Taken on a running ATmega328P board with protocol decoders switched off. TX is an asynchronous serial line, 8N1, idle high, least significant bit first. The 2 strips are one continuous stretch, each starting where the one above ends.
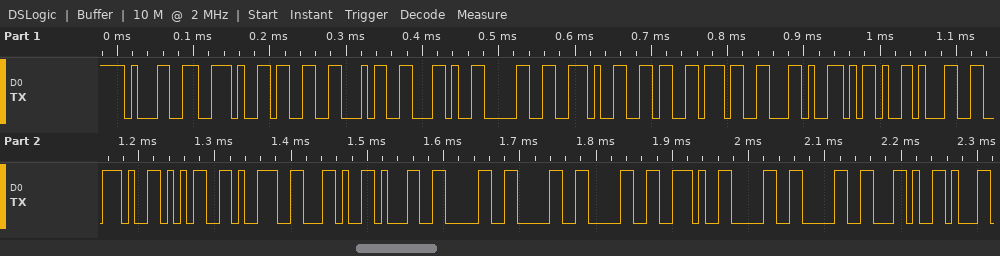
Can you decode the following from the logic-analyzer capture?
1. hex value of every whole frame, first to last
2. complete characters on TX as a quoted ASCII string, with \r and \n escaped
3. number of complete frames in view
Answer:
31 2E 33 34 2C 30 2E 36 37 2C 2D 31 2E 35 39 2C 31 30 30 30 2E 30 30 2C
"1.34,0.67,-1.59,1000.00,"
24
